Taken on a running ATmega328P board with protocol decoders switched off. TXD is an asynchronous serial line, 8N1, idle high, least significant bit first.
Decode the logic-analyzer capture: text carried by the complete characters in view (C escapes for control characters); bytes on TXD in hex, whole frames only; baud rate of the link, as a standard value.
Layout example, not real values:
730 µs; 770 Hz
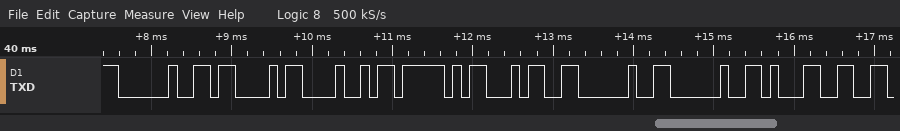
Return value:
" CH_4  1"; 0x20 0x43 0x48 0x5F 0x34 0x20 0x20 0x31; 9600 baud
